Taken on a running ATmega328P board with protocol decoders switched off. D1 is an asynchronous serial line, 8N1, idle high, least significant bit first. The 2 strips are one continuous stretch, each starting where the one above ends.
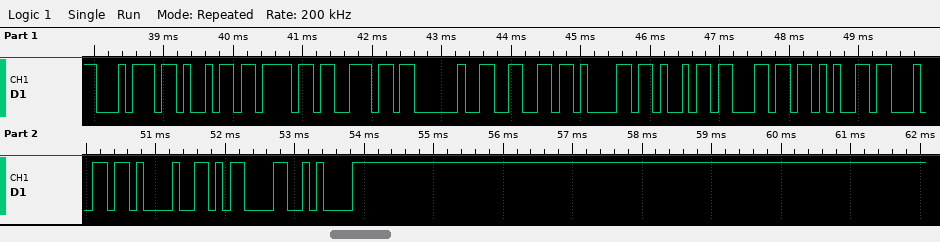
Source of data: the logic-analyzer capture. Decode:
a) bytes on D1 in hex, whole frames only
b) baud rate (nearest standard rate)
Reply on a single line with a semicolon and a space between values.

0x74 0x69 0x6F 0x6E 0x20 0x66 0x61 0x69 0x6C 0x65 0x64 0x21 0x0D 0x0A; 9600 baud
